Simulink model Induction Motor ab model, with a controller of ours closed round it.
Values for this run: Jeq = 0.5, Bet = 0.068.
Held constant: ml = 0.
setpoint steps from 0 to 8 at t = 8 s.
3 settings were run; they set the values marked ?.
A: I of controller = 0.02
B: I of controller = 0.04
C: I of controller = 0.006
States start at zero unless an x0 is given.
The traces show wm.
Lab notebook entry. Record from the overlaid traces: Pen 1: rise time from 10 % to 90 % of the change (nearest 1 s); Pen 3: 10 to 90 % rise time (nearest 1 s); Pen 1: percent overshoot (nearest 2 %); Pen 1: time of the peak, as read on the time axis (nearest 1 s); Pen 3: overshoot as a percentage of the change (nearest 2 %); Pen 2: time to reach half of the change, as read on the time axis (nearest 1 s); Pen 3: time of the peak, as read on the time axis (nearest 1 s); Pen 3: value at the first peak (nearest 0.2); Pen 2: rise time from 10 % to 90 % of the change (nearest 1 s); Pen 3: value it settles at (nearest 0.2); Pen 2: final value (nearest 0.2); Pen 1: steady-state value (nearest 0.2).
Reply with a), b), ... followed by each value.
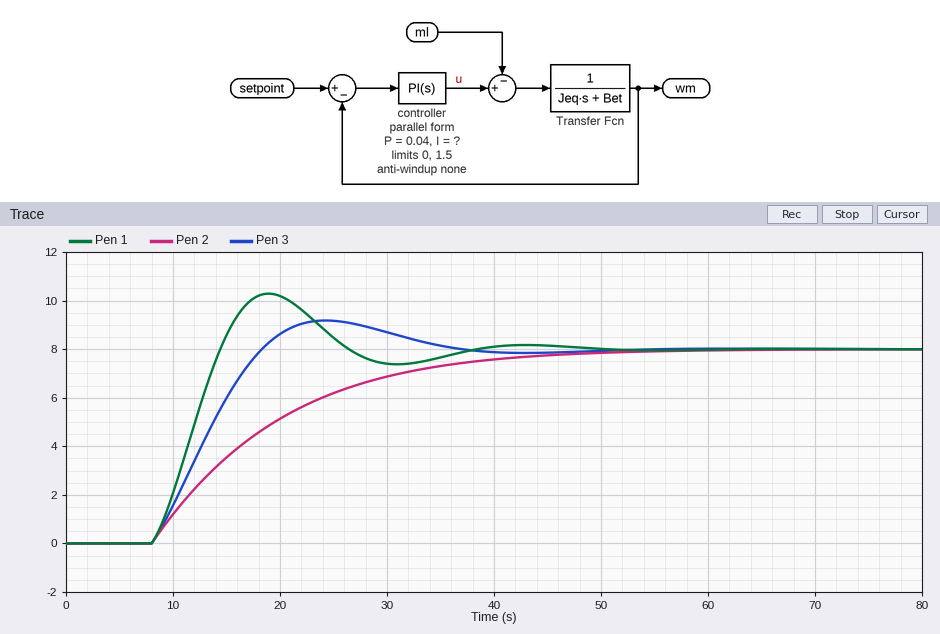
a) 5 s
b) 8 s
c) 28 %
d) 19 s
e) 14 %
f) 16 s
g) 24 s
h) 9.2
i) 24 s
j) 8.0
k) 8.0
l) 8.0
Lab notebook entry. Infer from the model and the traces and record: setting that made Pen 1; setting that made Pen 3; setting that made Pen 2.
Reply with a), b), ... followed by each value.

a) B
b) A
c) C
